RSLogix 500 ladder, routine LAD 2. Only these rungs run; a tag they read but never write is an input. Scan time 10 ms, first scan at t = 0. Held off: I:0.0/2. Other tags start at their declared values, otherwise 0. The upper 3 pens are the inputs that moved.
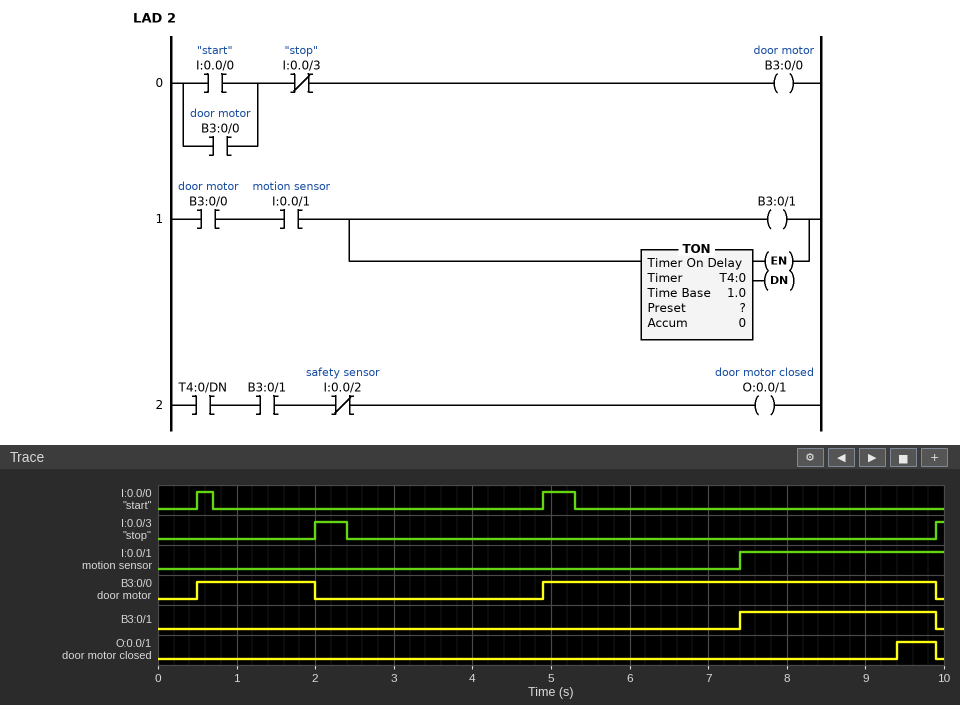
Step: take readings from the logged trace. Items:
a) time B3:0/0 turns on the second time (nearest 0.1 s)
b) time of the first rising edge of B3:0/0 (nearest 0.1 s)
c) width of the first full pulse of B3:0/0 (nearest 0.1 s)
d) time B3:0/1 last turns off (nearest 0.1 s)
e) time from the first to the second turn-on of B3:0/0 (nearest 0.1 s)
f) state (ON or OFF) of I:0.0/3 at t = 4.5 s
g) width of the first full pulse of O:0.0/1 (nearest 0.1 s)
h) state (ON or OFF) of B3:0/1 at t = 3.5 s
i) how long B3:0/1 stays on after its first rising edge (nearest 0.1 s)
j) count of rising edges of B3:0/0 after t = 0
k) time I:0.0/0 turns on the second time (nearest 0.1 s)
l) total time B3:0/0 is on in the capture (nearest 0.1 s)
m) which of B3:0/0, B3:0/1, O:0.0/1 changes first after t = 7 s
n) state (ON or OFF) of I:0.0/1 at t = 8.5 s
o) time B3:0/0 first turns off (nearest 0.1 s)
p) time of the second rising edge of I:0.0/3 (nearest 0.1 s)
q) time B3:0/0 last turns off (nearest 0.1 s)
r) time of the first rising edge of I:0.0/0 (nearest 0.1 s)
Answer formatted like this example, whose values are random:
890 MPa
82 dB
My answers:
4.9 s
0.5 s
1.5 s
9.9 s
4.4 s
OFF
0.5 s
OFF
2.5 s
2
4.9 s
6.5 s
B3:0/1
ON
2.0 s
9.9 s
9.9 s
0.5 s
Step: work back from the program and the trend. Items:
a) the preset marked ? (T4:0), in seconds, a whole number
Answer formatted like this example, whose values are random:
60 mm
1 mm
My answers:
2 s
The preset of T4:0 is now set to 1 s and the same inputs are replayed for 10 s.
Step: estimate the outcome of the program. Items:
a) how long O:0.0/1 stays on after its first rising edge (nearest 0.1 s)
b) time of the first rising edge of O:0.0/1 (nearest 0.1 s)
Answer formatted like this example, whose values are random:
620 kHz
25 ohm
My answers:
1.5 s
8.4 s
